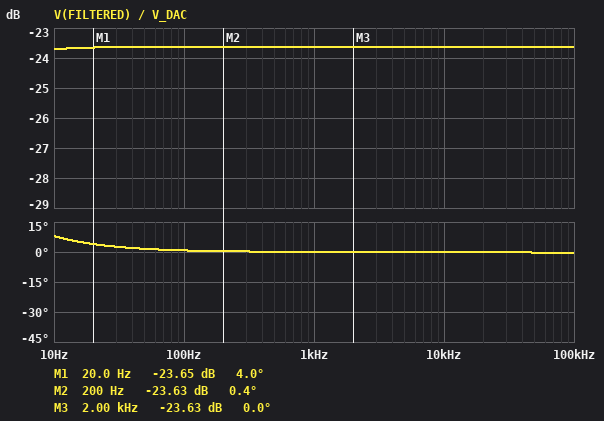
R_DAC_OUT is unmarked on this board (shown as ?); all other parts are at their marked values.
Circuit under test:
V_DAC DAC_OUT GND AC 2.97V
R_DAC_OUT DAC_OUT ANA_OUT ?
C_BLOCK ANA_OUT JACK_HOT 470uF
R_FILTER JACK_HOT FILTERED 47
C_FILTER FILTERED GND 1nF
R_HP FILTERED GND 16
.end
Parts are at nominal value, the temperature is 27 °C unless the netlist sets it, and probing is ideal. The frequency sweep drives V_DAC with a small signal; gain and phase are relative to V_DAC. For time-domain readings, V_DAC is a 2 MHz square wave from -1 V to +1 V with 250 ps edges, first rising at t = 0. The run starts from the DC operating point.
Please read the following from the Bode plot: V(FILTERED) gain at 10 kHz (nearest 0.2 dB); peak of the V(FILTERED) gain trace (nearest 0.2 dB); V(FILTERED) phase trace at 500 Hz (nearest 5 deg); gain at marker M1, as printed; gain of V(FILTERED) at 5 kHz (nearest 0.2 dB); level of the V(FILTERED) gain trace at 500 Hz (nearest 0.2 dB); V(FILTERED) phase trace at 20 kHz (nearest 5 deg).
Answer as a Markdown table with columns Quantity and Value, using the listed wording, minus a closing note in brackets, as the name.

| Quantity | Value |
|---|---|
| V(FILTERED) gain at 10 kHz | -23.6 dB |
| peak of the V(FILTERED) gain trace | -23.6 dB |
| V(FILTERED) phase trace at 500 Hz | 0 deg |
| gain at marker M1, as printed | -23.65 dB |
| gain of V(FILTERED) at 5 kHz | -23.6 dB |
| level of the V(FILTERED) gain trace at 500 Hz | -23.6 dB |
| V(FILTERED) phase trace at 20 kHz | 0 deg |
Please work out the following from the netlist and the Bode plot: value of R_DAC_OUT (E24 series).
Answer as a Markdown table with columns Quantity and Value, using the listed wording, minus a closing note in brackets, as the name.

| Quantity | Value |
|---|---|
| value of R_DAC_OUT | 180 Ω |
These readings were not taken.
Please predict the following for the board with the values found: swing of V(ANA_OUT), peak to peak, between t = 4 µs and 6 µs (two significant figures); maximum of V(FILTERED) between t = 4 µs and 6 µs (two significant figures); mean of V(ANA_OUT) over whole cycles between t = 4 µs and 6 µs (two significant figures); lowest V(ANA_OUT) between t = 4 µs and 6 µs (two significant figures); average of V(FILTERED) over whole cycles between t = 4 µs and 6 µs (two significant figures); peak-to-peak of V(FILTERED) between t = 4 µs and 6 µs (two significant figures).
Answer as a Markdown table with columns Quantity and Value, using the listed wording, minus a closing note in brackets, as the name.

| Quantity | Value |
|---|---|
| swing of V(ANA_OUT), peak to peak, between t = 4 µs and 6 µs | 520 mV |
| maximum of V(FILTERED) between t = 4 µs and 6 µs | 130 mV |
| mean of V(ANA_OUT) over whole cycles between t = 4 µs and 6 µs | -740 mV |
| lowest V(ANA_OUT) between t = 4 µs and 6 µs | -1.0 V |
| average of V(FILTERED) over whole cycles between t = 4 µs and 6 µs | 66 mV |
| peak-to-peak of V(FILTERED) between t = 4 µs and 6 µs | 130 mV |
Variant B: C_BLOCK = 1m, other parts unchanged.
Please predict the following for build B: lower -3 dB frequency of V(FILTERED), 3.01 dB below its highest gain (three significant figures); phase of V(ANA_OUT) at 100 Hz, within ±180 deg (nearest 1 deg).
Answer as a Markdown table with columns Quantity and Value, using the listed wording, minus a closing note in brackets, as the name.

| Quantity | Value |
|---|---|
| lower -3 dB frequency of V(FILTERED), 3.01 dB below its highest gain | 655 mHz |
| phase of V(ANA_OUT) at 100 Hz, within ±180 deg | -1 deg |
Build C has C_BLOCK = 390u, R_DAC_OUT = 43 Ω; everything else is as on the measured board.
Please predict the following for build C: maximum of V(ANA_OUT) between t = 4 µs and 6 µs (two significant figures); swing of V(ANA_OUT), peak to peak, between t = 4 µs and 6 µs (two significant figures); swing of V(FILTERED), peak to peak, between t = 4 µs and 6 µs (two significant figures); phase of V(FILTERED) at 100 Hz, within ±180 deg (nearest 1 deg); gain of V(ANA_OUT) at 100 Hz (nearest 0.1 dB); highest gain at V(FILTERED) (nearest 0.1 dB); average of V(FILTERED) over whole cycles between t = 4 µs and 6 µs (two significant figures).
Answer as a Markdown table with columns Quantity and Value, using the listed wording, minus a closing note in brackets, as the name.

| Quantity | Value |
|---|---|
| maximum of V(ANA_OUT) between t = 4 µs and 6 µs | 190 mV |
| swing of V(ANA_OUT), peak to peak, between t = 4 µs and 6 µs | 1.2 V |
| swing of V(FILTERED), peak to peak, between t = 4 µs and 6 µs | 300 mV |
| phase of V(FILTERED) at 100 Hz, within ±180 deg | 2 deg |
| gain of V(ANA_OUT) at 100 Hz | -4.5 dB |
| highest gain at V(FILTERED) | -16.4 dB |
| average of V(FILTERED) over whole cycles between t = 4 µs and 6 µs | 150 mV |
